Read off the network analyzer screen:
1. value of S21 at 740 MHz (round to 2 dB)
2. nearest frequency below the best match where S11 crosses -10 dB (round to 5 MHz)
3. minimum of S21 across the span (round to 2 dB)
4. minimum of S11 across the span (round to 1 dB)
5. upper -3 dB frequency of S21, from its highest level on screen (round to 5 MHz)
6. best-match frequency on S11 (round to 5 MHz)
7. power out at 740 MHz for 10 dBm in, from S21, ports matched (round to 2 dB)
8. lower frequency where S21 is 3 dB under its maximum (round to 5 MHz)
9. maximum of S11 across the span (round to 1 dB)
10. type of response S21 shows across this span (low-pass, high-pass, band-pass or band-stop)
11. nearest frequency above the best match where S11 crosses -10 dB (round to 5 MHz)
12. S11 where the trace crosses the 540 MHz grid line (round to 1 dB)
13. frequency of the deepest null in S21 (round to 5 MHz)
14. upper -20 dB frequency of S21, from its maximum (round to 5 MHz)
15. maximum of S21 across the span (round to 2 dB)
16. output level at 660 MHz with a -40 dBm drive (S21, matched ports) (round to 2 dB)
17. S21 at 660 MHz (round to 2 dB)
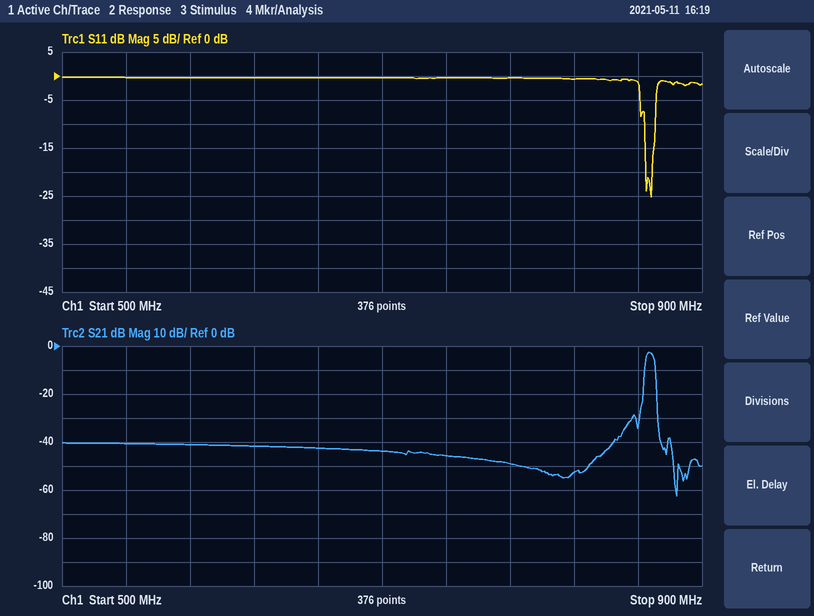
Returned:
-46 dB
865 MHz
-62 dB
-25 dB
870 MHz
870 MHz
-36 dBm
865 MHz
0 dB
band-pass
870 MHz
0 dB
885 MHz
870 MHz
-2 dB
-82 dBm
-42 dB
